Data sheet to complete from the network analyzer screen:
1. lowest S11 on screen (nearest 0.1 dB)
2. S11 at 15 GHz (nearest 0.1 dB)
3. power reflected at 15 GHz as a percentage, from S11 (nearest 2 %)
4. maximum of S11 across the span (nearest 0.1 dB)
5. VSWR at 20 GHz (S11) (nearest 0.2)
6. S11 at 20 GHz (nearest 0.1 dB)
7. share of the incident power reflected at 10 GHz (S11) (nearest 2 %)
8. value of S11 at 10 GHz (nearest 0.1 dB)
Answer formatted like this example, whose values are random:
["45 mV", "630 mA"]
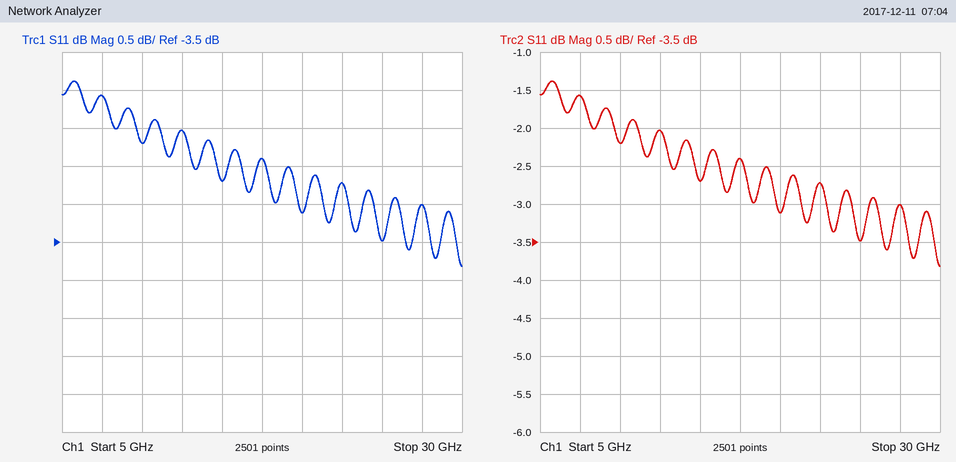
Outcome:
["-3.8 dB", "-2.7 dB", "54 %", "-1.4 dB", "5.6", "-3.1 dB", "60 %", "-2.2 dB"]
